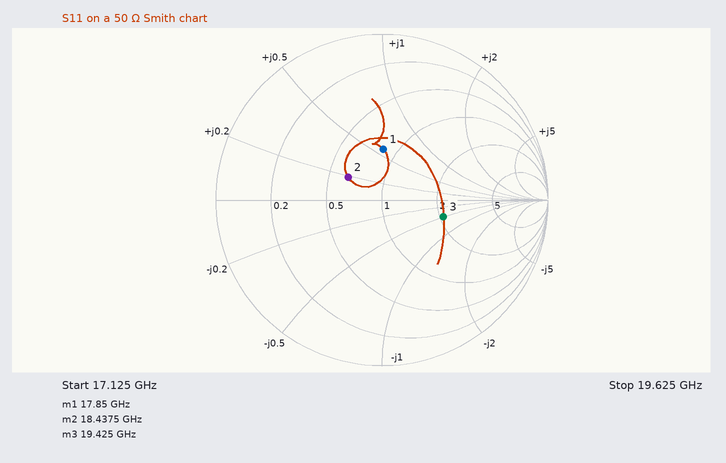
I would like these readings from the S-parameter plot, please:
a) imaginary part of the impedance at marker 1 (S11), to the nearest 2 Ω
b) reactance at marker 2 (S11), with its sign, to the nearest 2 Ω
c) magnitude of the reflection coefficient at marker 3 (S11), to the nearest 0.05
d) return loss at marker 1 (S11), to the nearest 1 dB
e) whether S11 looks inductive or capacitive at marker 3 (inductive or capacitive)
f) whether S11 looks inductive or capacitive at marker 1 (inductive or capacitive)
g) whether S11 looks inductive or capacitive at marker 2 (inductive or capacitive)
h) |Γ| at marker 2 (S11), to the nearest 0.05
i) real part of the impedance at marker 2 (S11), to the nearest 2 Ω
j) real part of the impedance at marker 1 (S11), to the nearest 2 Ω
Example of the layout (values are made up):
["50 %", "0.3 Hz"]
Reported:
["+28 Ω", "+10 Ω", "0.40", "10 dB", "capacitive", "inductive", "inductive", "0.25", "32 Ω", "42 Ω"]
